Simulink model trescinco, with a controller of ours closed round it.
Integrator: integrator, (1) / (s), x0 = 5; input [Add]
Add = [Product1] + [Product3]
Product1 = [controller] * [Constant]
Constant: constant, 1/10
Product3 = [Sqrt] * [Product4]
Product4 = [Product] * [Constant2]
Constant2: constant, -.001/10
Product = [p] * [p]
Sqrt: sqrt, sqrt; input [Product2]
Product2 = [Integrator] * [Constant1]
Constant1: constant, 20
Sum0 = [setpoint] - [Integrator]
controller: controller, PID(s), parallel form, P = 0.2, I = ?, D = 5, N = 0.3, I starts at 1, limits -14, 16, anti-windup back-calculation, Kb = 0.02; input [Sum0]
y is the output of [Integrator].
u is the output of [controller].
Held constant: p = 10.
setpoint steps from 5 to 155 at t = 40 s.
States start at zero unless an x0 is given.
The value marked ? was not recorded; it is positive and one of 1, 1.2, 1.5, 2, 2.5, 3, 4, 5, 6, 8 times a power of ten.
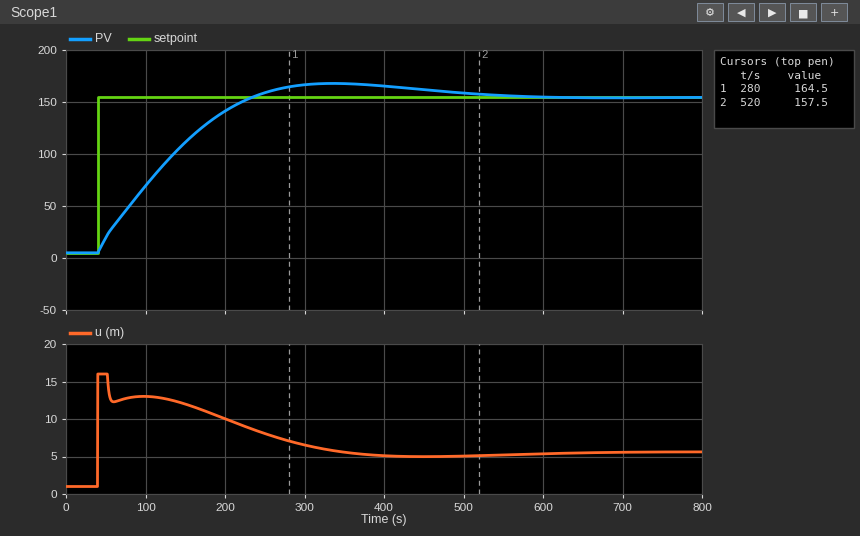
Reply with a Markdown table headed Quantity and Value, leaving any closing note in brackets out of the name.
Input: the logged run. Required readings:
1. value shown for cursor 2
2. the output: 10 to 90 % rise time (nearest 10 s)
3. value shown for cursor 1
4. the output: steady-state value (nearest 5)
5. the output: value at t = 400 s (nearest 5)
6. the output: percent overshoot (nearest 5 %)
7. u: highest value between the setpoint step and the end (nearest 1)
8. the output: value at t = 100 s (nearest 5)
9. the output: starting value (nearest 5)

| Quantity | Value |
|---|---|
| value shown for cursor 2 | 157.5 |
| the output: 10 to 90 % rise time | 150 s |
| value shown for cursor 1 | 164.5 |
| the output: steady-state value | 155 |
| the output: value at t = 400 s | 165 |
| the output: percent overshoot | 10 % |
| u: highest value between the setpoint step and the end | 16 |
| the output: value at t = 100 s | 70 |
| the output: starting value | 5 |
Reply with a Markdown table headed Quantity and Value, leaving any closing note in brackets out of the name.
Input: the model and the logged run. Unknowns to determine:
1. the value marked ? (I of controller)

| Quantity | Value |
|---|---|
| the value marked ? | 0.002 |
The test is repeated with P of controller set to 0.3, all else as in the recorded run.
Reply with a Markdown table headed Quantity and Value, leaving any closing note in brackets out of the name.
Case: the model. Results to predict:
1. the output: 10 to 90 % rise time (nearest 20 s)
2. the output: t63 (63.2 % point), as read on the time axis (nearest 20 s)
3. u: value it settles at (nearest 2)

| Quantity | Value |
|---|---|
| the output: 10 to 90 % rise time | 160 s |
| the output: t63 (63.2 % point), as read on the time axis | 120 s |
| u: value it settles at | 6 |
